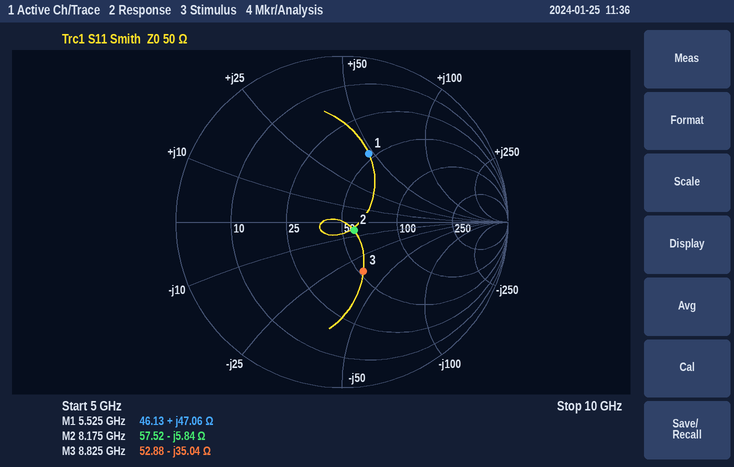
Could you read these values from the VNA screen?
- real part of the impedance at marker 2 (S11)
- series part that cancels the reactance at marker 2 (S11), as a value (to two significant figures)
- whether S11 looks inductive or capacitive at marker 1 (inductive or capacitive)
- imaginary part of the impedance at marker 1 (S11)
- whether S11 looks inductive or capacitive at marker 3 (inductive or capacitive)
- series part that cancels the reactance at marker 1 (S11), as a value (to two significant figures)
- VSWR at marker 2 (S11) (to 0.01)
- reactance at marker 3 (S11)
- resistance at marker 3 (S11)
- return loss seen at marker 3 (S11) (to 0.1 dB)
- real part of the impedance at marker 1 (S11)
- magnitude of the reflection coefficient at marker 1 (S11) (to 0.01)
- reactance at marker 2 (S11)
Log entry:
57.52 Ω
110 pH
inductive
+47.06 Ω
capacitive
610 fF
1.19
-35.04 Ω
52.88 Ω
9.8 dB
46.13 Ω
0.44
-5.84 Ω
